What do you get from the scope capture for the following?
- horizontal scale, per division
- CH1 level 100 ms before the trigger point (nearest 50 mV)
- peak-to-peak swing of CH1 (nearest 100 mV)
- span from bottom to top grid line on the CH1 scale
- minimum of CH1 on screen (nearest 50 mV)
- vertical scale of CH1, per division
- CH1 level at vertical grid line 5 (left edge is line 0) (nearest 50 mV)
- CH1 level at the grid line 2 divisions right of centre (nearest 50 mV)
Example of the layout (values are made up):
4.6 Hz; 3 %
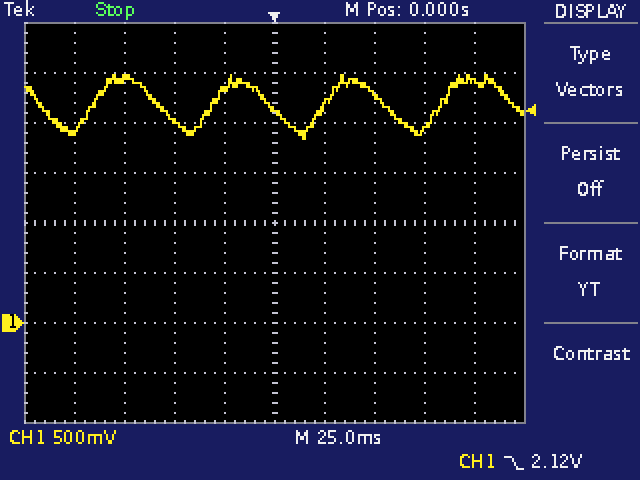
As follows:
25 ms; 1.90 V; 600 mV; 4 V; 1.85 V; 500 mV; 2.10 V; 2.30 V
